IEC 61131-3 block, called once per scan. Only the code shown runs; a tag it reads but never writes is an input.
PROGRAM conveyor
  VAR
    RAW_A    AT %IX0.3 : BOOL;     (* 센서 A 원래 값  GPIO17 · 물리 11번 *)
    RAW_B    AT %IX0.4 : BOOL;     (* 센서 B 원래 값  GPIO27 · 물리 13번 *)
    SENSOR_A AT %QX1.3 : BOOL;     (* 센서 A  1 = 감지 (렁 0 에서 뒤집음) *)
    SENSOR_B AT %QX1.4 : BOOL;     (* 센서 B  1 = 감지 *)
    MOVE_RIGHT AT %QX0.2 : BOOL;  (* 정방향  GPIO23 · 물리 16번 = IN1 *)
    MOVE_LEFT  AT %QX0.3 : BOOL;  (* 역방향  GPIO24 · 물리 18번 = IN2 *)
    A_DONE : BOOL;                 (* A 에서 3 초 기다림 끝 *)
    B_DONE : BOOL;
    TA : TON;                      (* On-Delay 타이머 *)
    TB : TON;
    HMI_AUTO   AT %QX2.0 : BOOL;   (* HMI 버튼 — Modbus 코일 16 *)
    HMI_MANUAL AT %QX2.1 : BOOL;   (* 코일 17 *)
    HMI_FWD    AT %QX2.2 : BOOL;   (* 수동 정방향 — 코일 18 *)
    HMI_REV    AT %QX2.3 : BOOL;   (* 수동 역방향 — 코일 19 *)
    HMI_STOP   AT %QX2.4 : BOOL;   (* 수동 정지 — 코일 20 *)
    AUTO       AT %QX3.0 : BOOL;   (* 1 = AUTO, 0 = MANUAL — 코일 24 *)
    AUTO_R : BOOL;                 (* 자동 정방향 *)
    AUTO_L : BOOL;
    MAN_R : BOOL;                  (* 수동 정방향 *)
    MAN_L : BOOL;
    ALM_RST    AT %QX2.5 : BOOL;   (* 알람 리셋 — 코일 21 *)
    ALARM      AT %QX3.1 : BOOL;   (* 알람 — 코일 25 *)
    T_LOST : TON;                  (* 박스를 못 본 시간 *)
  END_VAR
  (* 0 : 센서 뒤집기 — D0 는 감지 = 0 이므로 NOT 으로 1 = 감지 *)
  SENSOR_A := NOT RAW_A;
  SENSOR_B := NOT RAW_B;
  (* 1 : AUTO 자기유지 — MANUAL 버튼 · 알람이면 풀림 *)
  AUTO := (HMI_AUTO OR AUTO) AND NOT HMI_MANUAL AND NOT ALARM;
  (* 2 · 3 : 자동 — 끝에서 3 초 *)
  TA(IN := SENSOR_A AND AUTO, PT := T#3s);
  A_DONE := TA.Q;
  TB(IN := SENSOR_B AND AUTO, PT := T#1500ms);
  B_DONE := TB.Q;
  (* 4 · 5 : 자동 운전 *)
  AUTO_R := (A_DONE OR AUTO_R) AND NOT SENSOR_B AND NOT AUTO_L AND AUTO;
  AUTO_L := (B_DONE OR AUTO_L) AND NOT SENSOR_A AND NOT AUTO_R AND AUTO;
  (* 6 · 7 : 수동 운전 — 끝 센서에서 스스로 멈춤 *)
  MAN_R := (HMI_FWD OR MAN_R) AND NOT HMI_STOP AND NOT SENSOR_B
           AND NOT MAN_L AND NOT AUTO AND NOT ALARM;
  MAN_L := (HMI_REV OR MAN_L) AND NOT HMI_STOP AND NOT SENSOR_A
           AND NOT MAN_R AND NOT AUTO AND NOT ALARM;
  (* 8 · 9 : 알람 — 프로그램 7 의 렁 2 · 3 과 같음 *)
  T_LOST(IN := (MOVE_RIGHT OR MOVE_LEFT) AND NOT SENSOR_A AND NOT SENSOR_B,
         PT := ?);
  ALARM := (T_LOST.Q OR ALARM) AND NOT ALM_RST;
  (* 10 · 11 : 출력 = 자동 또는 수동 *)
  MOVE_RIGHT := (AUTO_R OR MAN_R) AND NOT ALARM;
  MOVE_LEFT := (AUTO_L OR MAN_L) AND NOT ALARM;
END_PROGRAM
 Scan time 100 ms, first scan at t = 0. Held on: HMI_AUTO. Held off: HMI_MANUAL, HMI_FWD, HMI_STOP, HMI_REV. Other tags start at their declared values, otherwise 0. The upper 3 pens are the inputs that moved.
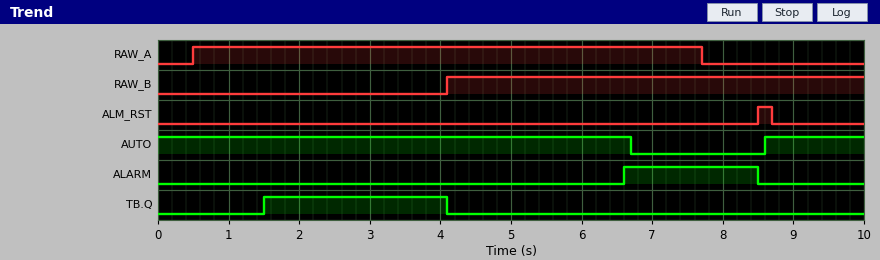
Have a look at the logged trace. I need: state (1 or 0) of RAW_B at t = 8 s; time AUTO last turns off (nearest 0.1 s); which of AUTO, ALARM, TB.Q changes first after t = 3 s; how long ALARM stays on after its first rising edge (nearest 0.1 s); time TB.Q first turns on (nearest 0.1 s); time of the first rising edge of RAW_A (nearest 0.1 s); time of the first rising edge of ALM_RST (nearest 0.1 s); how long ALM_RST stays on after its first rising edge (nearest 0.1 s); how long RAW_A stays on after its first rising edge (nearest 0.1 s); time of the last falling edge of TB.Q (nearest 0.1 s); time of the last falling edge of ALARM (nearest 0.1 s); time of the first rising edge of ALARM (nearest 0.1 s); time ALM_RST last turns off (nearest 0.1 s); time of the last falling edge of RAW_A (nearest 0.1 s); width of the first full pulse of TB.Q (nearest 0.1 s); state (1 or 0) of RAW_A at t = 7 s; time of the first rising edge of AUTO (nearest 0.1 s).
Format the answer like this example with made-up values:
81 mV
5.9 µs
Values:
1
6.7 s
TB.Q
1.9 s
1.5 s
0.5 s
8.5 s
0.2 s
7.2 s
4.1 s
8.5 s
6.6 s
8.7 s
7.7 s
2.6 s
1
8.6 s
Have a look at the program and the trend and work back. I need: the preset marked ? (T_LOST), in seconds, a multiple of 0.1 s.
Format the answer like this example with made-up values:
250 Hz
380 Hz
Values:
2.5 s
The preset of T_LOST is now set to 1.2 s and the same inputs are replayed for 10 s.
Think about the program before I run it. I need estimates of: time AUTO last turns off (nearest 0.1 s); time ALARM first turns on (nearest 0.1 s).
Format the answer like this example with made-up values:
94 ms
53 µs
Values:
5.4 s
5.3 s
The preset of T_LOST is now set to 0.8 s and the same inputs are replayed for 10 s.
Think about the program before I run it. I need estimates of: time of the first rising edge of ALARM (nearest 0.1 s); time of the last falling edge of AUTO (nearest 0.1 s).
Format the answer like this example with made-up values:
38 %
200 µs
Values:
4.9 s
5.0 s
